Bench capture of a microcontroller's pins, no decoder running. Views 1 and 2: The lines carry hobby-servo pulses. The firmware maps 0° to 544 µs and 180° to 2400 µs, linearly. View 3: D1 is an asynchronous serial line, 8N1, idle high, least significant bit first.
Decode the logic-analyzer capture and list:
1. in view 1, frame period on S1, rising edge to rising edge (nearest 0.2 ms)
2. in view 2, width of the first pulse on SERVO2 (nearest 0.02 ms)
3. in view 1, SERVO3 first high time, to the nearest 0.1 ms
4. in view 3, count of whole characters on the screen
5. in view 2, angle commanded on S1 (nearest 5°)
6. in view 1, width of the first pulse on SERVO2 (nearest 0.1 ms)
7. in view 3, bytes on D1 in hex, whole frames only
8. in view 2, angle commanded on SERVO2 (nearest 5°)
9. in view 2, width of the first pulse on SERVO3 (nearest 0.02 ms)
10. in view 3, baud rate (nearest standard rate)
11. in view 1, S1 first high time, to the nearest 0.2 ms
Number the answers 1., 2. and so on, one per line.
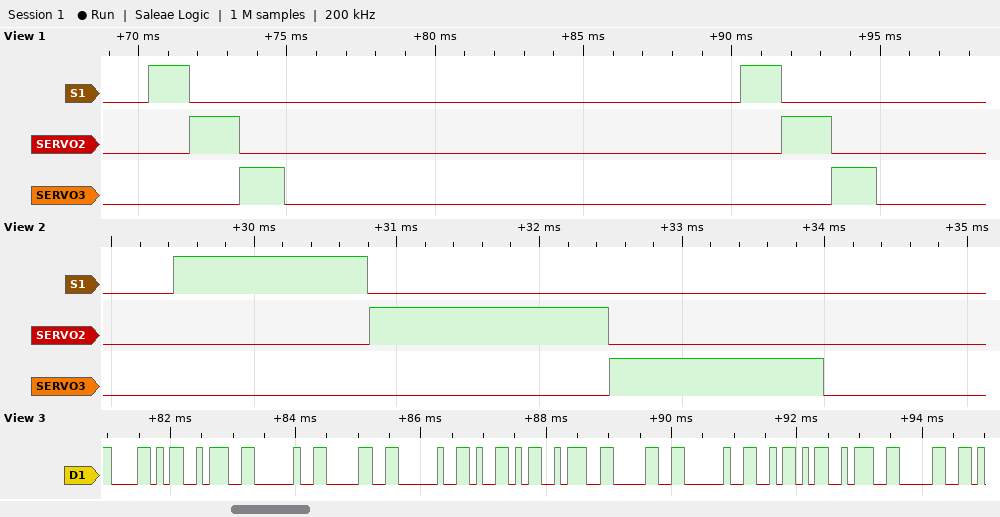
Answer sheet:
1. 20.0 ms
2. 1.68 ms
3. 1.5 ms
4. 12
5. 80°
6. 1.7 ms
7. 58 3A 20 30 20 59 3A 30 20 5A 3A 30
8. 110°
9. 1.50 ms
10. 9600 baud
11. 1.4 ms
